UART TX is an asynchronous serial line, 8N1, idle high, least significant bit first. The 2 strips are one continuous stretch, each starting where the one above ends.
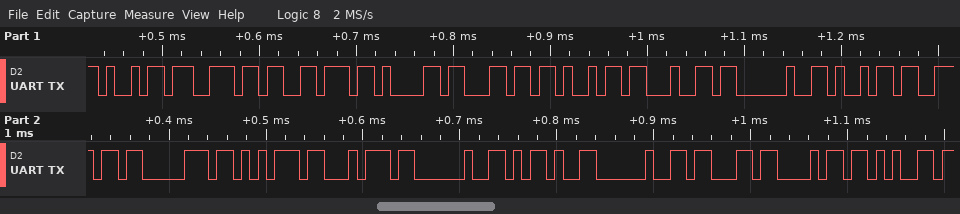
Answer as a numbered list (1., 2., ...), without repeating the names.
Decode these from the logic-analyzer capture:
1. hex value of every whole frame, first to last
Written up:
1. 0x69 0x6E 0x76 0x61 0x6C 0x69 0x64 0x20 0x69 0x6E 0x70 0x75 0x74 0x20 0x2D 0x20 0x63 0x68 0x65
